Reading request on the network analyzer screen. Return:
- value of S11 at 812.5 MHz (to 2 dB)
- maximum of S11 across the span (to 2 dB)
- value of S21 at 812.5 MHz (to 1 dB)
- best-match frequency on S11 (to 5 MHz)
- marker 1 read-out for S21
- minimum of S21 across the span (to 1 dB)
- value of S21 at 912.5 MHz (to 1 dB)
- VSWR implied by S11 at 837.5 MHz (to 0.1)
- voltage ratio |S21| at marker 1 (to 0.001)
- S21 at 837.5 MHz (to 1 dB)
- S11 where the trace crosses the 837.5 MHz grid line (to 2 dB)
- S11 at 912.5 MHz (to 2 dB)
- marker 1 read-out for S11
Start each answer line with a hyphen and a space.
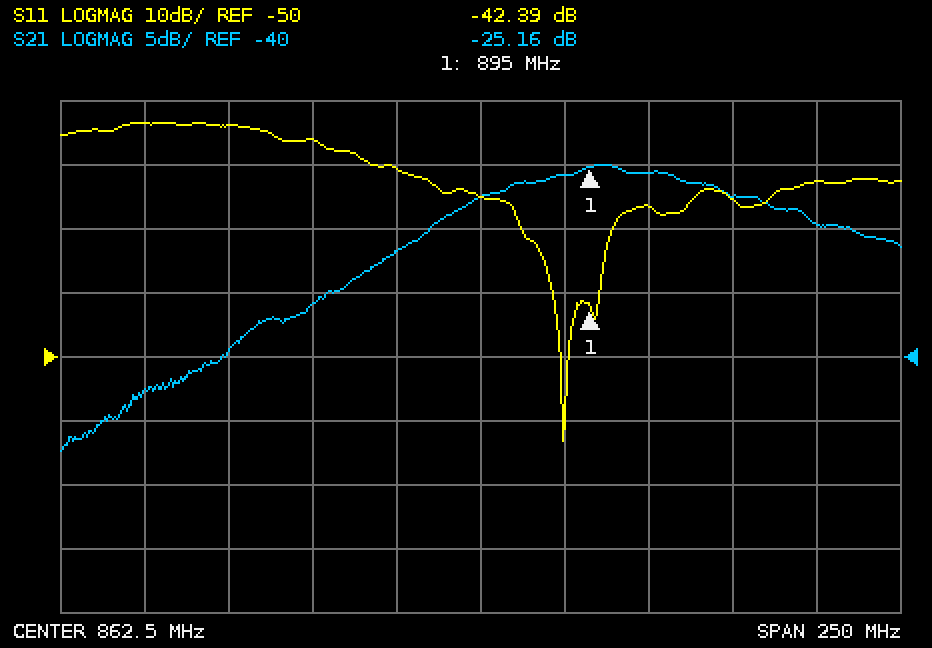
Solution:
- -16 dB
- -14 dB
- -36 dB
- 885 MHz
- -25.16 dB
- -47 dB
- -26 dB
- 1.2
- 0.055
- -32 dB
- -20 dB
- -26 dB
- -42.39 dB
